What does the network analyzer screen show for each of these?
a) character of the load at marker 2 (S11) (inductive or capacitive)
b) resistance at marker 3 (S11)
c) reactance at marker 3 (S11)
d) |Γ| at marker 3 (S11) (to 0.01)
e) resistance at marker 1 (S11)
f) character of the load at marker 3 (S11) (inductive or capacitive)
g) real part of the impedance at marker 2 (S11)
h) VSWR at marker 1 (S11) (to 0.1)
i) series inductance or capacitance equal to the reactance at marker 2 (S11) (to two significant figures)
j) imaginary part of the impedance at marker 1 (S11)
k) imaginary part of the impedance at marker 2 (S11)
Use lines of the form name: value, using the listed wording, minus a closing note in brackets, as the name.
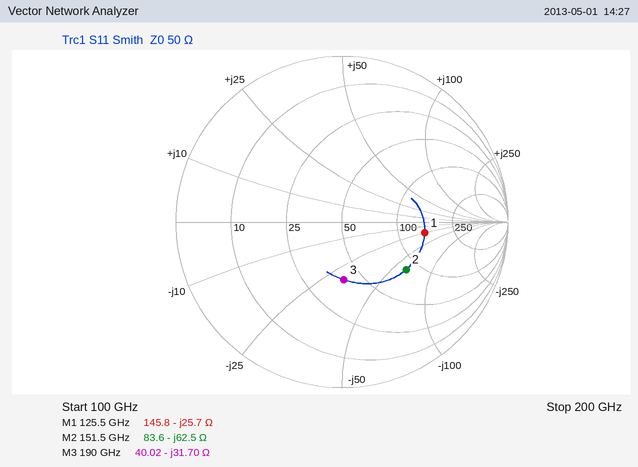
character of the load at marker 2 (S11): capacitive
resistance at marker 3: 40.02 Ω
reactance at marker 3: -31.70 Ω
|Γ| at marker 3 (S11): 0.35
resistance at marker 1: 145.8 Ω
character of the load at marker 3 (S11): capacitive
real part of the impedance at marker 2: 83.6 Ω
VSWR at marker 1 (S11): 3.0
series inductance or capacitance equal to the reactance at marker 2 (S11): 17 fF
imaginary part of the impedance at marker 1: -25.7 Ω
imaginary part of the impedance at marker 2: -62.5 Ω
